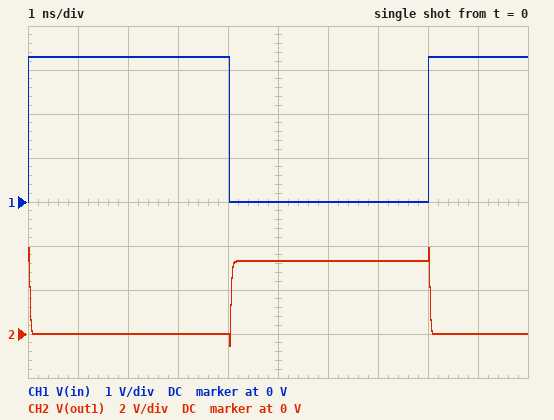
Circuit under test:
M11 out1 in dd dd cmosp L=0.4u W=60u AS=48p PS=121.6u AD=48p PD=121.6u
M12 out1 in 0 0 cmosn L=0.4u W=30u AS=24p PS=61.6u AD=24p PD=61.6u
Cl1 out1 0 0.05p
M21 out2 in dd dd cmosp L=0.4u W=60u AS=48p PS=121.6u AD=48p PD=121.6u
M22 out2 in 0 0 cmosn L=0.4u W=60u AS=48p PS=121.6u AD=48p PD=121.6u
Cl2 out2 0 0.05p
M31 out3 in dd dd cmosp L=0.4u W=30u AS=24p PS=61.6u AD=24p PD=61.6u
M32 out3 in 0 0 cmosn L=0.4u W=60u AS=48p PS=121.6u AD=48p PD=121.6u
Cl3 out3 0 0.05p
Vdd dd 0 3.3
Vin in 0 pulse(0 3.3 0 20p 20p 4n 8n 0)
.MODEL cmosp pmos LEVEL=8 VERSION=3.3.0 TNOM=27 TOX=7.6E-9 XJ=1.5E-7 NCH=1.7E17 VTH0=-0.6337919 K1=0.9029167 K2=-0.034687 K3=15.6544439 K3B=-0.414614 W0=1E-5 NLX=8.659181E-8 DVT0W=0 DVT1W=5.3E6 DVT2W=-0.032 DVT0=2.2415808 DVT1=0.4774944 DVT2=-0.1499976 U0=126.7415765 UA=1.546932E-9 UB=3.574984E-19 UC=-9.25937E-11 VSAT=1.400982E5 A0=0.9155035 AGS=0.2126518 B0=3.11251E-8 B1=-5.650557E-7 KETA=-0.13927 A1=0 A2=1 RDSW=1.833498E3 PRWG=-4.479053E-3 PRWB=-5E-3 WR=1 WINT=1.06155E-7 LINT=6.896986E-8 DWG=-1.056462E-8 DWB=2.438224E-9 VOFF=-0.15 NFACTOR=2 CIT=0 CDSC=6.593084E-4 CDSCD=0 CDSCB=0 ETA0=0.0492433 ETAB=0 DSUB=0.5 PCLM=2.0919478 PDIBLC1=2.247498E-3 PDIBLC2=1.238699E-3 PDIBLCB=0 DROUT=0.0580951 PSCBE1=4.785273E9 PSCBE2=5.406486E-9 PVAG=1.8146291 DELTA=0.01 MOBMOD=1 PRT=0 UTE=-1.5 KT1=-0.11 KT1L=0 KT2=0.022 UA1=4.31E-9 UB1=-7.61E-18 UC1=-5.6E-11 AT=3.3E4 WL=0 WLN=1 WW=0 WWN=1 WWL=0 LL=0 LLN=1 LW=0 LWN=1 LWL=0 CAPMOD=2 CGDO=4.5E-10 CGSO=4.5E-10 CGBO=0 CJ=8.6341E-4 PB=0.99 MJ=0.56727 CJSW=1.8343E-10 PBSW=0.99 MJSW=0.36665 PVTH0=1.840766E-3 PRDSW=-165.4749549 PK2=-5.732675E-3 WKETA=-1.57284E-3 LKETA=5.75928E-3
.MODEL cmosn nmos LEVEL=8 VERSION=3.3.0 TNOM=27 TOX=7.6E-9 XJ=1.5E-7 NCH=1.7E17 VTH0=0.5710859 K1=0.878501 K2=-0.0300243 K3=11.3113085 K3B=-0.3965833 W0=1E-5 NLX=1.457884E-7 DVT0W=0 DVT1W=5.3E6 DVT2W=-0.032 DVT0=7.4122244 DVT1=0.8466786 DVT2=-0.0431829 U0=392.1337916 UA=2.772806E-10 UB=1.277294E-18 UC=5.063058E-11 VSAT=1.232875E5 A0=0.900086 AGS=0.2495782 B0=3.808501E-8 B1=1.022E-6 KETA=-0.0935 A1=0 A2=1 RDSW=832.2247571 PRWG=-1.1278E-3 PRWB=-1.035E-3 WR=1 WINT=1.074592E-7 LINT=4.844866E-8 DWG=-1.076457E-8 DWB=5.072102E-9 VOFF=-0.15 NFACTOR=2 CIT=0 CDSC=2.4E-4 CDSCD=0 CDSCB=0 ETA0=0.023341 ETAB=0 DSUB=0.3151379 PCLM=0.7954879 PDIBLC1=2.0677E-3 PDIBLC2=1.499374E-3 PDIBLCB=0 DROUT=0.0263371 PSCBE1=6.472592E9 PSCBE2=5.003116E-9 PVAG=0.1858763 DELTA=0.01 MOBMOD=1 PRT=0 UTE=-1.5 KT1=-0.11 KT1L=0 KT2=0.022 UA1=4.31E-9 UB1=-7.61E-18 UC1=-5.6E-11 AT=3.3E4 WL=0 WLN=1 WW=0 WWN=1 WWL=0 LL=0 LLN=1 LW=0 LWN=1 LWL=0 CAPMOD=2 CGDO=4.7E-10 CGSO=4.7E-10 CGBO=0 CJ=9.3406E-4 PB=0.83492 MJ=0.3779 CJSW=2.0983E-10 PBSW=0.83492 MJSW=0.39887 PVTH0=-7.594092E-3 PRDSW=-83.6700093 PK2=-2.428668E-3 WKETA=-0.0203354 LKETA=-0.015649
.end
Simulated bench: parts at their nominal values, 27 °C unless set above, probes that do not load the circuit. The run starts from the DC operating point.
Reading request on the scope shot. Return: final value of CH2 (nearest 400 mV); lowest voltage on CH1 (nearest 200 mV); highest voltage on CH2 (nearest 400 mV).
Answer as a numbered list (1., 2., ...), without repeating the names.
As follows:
1. 0 V
2. 0 V
3. 4.0 V
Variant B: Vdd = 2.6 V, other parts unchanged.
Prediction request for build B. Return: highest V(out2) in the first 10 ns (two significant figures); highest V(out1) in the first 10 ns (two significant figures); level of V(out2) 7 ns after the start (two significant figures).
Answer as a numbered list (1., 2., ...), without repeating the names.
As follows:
1. 3.2 V
2. 3.3 V
3. 2.6 V
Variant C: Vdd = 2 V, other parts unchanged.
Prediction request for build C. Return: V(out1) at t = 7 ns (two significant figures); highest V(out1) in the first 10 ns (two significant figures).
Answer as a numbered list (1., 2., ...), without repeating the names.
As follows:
1. 2.0 V
2. 2.7 V
